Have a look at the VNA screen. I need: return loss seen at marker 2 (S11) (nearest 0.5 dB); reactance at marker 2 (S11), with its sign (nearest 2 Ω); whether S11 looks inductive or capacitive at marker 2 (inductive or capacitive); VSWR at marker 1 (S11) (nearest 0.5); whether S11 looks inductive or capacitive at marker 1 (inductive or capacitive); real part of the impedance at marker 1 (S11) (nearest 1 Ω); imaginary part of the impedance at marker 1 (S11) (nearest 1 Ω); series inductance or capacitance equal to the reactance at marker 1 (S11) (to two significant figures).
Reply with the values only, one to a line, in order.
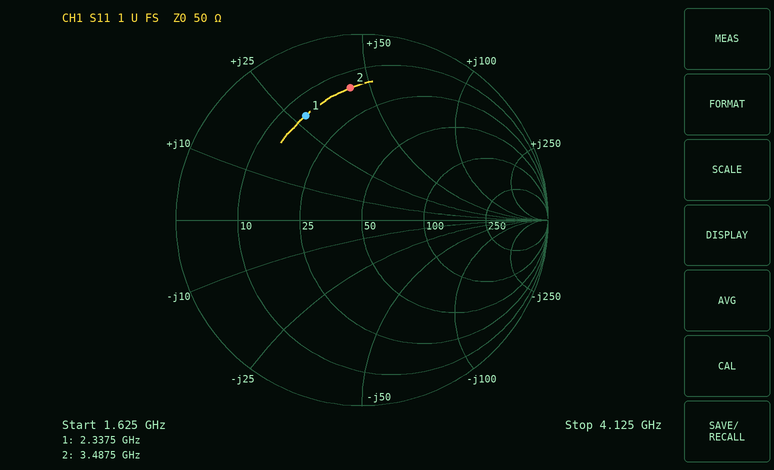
3.0 dB
+44 Ω
inductive
4.5
inductive
15 Ω
+28 Ω
1.9 nH
